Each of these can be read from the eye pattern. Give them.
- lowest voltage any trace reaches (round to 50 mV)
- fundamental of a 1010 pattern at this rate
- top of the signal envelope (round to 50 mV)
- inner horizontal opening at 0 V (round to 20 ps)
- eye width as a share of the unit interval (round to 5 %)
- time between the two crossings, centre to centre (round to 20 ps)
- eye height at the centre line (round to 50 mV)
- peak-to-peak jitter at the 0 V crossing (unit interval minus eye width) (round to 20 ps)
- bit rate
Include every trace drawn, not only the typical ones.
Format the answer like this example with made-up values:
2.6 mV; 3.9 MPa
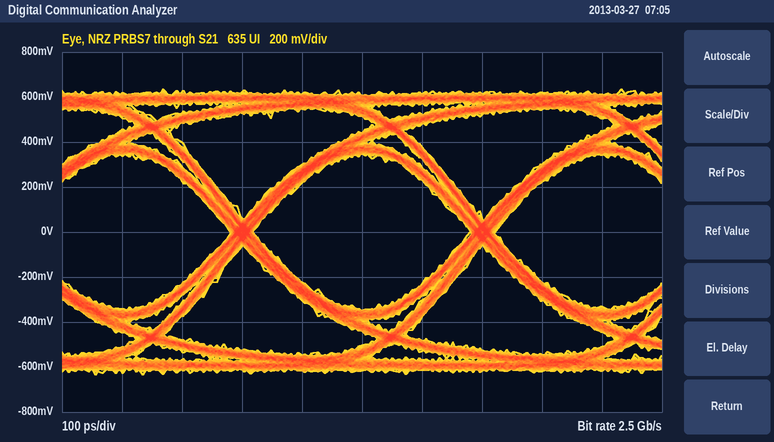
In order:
-650 mV; 1.25 GHz; 650 mV; 360 ps; 90 %; 400 ps; 700 mV; 40 ps; 2.5 Gb/s
